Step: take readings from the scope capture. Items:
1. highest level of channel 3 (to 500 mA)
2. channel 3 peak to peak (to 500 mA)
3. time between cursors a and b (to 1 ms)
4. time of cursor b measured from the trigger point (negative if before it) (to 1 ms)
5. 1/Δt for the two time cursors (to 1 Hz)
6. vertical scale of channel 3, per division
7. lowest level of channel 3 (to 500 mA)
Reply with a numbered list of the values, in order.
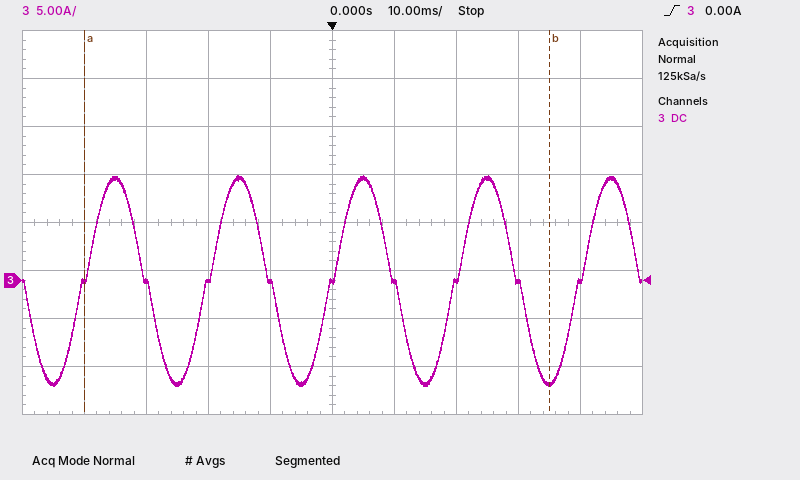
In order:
1. 11.0 A
2. 22.0 A
3. 75 ms
4. +35 ms
5. 13 Hz
6. 5 A
7. -11.0 A
